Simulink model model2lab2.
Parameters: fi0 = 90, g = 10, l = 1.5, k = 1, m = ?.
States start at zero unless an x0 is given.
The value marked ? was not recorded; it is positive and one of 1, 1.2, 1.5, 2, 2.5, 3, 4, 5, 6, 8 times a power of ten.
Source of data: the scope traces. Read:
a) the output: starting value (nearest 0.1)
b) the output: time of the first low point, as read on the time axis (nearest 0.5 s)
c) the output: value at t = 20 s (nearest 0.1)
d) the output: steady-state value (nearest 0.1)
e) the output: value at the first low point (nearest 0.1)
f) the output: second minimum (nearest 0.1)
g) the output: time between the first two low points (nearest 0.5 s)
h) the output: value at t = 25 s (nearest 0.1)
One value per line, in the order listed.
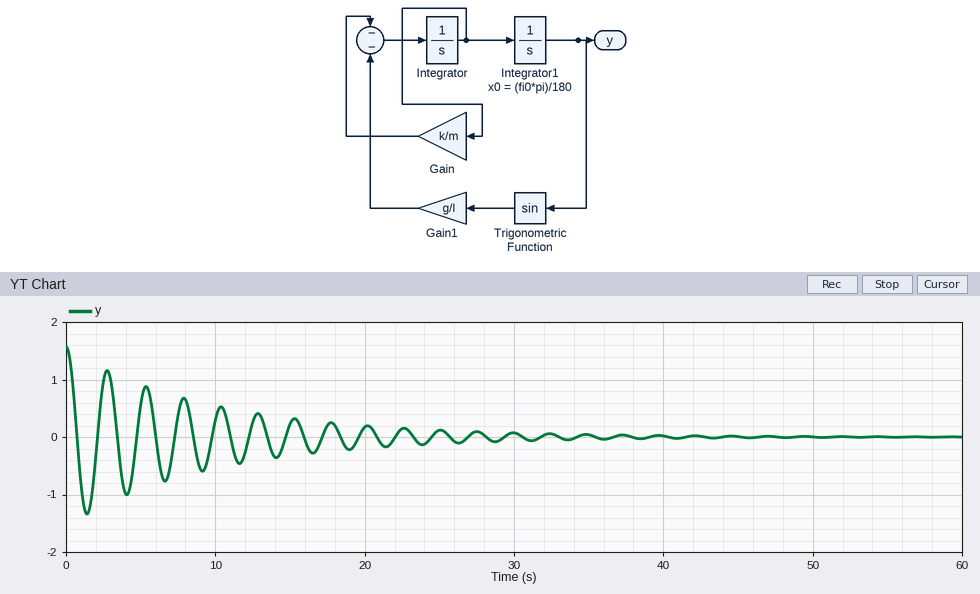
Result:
1.6
1.5 s
0.2
0.0
-1.3
-1.0
2.5 s
0.1
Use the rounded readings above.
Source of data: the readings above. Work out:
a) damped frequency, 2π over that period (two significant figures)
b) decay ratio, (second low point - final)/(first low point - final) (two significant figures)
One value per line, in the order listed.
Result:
2.5 rad/s
0.77
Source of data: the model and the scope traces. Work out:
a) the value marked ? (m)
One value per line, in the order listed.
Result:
5
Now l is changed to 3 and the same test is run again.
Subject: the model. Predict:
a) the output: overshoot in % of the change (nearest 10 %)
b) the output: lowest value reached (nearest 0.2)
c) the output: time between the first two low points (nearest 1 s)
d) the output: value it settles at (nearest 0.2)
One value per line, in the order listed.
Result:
80 %
-1.2
4 s
0.0
